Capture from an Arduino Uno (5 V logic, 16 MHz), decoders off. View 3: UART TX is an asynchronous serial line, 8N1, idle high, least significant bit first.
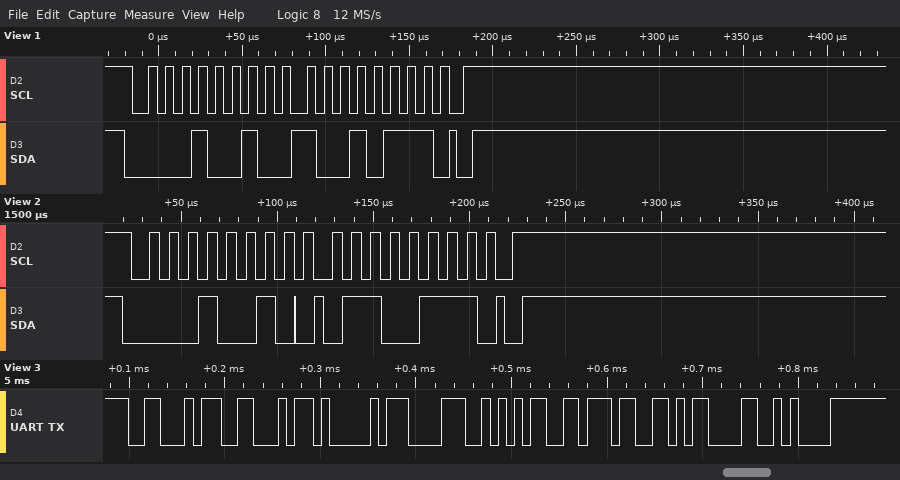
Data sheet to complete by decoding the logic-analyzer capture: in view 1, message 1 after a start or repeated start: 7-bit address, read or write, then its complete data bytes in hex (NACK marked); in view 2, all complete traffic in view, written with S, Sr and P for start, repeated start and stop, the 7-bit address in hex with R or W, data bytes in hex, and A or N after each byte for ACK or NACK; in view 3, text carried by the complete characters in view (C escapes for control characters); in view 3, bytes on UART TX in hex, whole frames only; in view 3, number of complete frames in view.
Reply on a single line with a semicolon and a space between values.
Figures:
0x09 write: 97; S 09W A 67 A P; "FFA857\r\n"; 46 46 41 38 35 37 0D 0A; 8
